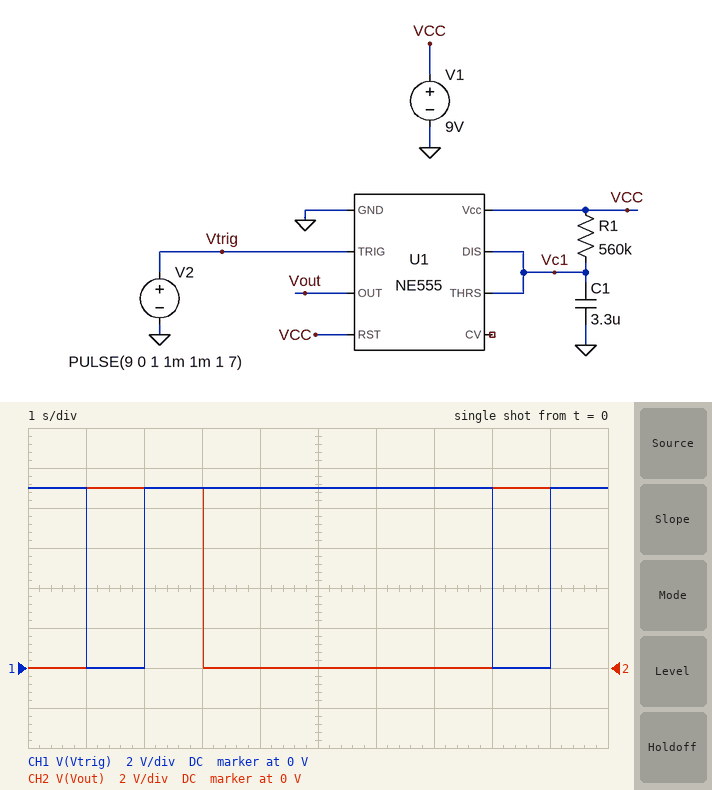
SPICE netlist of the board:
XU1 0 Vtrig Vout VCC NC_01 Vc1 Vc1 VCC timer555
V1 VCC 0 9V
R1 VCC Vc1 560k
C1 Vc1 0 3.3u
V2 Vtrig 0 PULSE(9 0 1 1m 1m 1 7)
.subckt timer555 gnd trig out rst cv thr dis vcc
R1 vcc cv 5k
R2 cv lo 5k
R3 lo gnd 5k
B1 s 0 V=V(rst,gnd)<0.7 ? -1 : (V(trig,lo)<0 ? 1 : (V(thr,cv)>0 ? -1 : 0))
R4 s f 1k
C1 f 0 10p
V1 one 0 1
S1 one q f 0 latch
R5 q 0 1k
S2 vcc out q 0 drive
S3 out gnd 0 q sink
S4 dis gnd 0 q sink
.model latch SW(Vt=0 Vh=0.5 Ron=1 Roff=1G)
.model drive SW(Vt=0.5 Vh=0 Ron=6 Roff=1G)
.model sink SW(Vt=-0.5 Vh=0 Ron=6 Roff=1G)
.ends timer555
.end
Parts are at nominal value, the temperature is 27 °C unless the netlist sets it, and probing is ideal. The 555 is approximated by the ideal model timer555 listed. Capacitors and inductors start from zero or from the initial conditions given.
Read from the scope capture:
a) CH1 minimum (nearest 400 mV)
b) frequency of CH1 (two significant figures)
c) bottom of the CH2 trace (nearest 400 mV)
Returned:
0 V
140 mHz
0 V
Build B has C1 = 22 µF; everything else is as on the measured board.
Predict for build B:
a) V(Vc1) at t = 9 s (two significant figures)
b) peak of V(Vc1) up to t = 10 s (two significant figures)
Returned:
4.3 V
4.7 V
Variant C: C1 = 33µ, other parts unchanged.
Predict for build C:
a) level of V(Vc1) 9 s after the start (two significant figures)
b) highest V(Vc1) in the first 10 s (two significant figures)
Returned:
3.2 V
3.5 V
